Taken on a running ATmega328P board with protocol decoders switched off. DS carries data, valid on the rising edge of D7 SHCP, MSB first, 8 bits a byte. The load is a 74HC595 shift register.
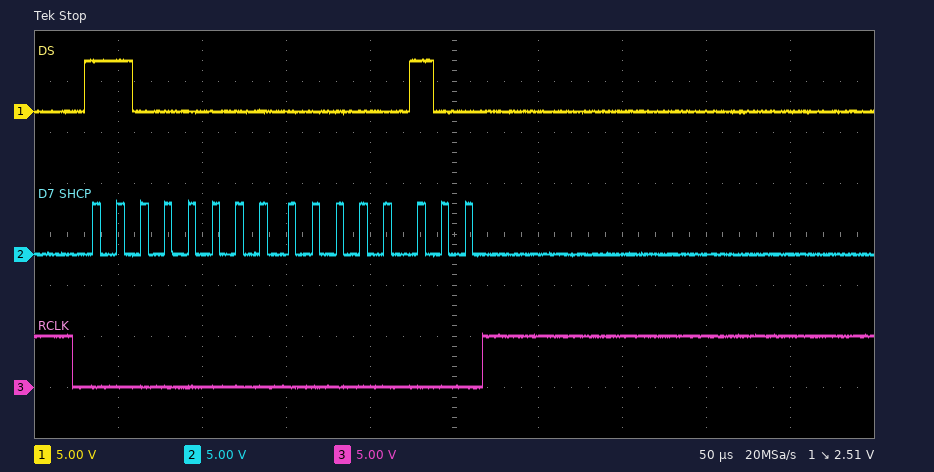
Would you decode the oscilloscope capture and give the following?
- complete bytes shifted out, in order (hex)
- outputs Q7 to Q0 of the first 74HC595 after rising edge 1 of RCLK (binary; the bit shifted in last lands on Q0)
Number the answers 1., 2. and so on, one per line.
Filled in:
1. C0 04
2. 00000100
